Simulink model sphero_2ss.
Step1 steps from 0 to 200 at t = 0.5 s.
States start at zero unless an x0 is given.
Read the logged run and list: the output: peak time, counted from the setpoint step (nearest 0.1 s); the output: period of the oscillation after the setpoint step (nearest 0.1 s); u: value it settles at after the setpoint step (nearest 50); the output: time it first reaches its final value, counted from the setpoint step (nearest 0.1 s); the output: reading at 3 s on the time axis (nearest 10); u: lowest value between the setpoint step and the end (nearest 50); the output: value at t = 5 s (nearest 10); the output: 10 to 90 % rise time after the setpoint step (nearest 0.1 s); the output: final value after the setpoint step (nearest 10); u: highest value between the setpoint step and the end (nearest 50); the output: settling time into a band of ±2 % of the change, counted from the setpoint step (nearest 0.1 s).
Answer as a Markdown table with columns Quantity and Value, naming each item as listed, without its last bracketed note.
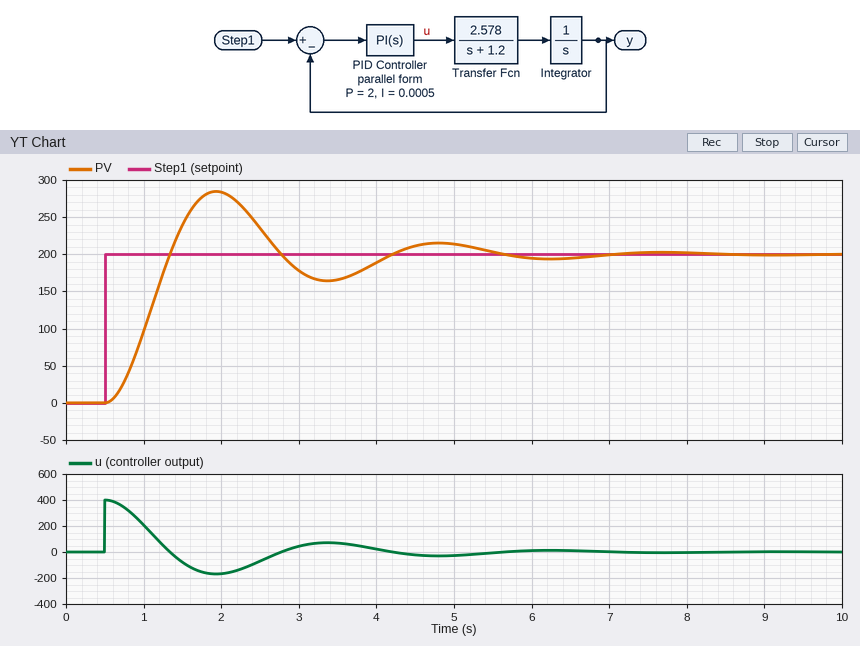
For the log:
| Quantity | Value |
|---|---|
| the output: peak time, counted from the setpoint step | 1.4 s |
| the output: period of the oscillation after the setpoint step | 2.9 s |
| u: value it settles at after the setpoint step | 0 |
| the output: time it first reaches its final value, counted from the setpoint step | 0.8 s |
| the output: reading at 3 s on the time axis | 180 |
| u: lowest value between the setpoint step and the end | -150 |
| the output: value at t = 5 s | 210 |
| the output: 10 to 90 % rise time after the setpoint step | 0.6 s |
| the output: final value after the setpoint step | 200 |
| u: highest value between the setpoint step and the end | 400 |
| the output: settling time into a band of ±2 % of the change, counted from the setpoint step | 6.2 s |
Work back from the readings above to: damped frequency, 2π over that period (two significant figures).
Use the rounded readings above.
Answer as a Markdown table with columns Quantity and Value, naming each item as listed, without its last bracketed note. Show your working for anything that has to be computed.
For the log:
| Quantity | Value |
|---|---|
| damped frequency, 2π over that period | 2π / 2.9 = 2.2 rad/s |
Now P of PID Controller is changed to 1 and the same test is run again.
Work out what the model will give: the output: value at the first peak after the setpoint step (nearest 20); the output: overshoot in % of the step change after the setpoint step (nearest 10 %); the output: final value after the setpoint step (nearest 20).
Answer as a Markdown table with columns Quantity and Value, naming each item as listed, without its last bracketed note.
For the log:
| Quantity | Value |
|---|---|
| the output: value at the first peak after the setpoint step | 260 |
| the output: overshoot in % of the step change after the setpoint step | 30 % |
| the output: final value after the setpoint step | 200 |
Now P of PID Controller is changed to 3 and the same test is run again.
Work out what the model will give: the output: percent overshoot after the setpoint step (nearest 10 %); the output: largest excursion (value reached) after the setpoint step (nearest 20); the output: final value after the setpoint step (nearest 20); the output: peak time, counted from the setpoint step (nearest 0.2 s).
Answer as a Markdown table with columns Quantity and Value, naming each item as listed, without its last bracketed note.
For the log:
| Quantity | Value |
|---|---|
| the output: percent overshoot after the setpoint step | 50 % |
| the output: largest excursion (value reached) after the setpoint step | 300 |
| the output: final value after the setpoint step | 200 |
| the output: peak time, counted from the setpoint step | 1.2 s |
